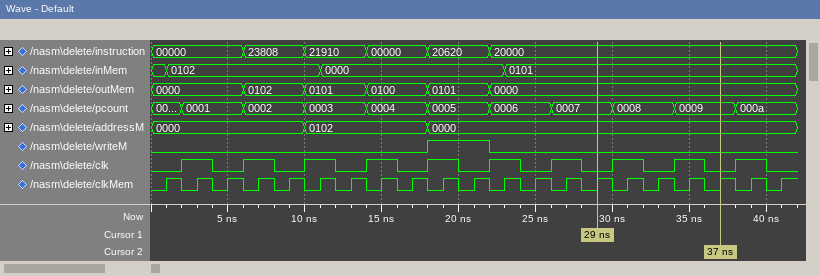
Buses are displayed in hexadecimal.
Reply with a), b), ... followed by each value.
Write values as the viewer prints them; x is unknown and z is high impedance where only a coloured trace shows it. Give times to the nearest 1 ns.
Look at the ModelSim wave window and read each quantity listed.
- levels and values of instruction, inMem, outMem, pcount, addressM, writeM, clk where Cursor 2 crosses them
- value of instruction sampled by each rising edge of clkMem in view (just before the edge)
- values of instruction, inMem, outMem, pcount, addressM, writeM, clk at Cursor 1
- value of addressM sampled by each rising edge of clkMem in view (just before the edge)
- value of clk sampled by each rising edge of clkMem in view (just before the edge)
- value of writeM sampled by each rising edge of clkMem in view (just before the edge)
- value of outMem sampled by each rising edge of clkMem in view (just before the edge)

a) instruction=20000, inMem=0101, outMem=0000, pcount=0009, addressM=0000, writeM=0, clk=0
b) 00000, 00000, 00000, 23808, 23808, 21910, 21910, 00000, 00000, 20620, 20620, 20000, 20000, 20000, 20000, 20000, 20000, 20000, 20000, 20000, 20000
c) instruction=20000, inMem=0101, outMem=0000, pcount=0007, addressM=0000, writeM=0, clk=0
d) 0000, 0000, 0000, 0000, 0000, 0102, 0102, 0102, 0102, 0000, 0000, 0000, 0000, 0000, 0000, 0000, 0000, 0000, 0000, 0000, 0000
e) 0 1 0 1 0 1 0 1 0 1 0 1 0 1 0 1 0 1 0 1 0
f) 0 0 0 0 0 0 0 0 0 1 1 0 0 0 0 0 0 0 0 0 0
g) 0000, 0000, 0000, 0102, 0102, 0101, 0101, 0100, 0100, 0101, 0101, 0000, 0000, 0000, 0000, 0000, 0000, 0000, 0000, 0000, 0000
